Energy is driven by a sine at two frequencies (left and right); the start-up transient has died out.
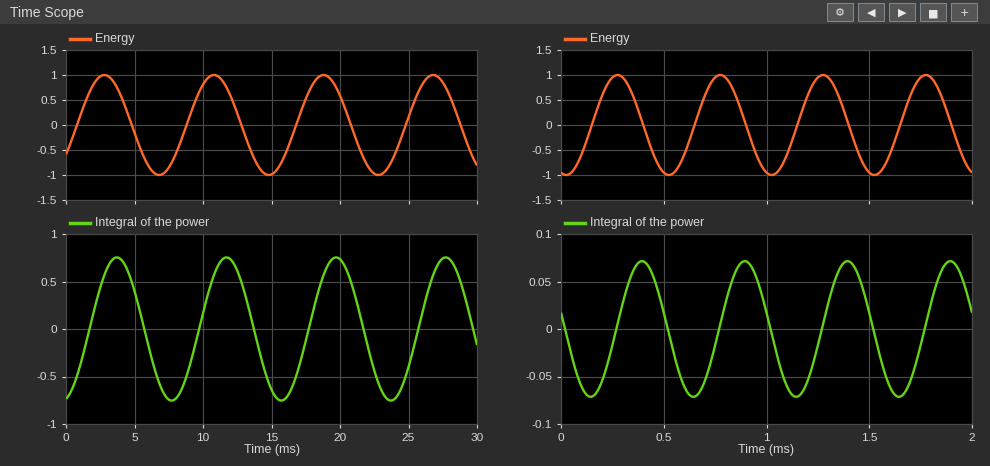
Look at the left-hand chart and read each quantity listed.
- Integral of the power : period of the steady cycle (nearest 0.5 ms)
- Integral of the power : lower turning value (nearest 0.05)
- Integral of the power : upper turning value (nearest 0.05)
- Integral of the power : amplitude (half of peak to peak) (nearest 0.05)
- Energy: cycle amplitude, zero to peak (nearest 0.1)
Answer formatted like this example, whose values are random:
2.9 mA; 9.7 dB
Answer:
8.0 ms; -0.75; 0.75; 0.75; 1.0
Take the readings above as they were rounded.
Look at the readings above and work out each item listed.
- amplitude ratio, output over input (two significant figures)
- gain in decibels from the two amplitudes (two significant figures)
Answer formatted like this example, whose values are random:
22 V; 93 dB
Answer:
0.75; -2.5 dB
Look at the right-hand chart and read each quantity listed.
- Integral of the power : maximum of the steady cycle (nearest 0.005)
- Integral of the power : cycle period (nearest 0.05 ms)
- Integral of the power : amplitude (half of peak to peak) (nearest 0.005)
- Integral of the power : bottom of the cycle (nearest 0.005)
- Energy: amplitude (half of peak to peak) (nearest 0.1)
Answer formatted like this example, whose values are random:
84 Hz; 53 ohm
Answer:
0.070; 0.50 ms; 0.070; -0.070; 1.0
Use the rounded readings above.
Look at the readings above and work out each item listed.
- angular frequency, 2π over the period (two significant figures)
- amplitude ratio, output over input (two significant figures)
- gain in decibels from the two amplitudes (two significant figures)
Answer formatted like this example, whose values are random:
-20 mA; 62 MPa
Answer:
13 rad/ms; 0.070; -23 dB
